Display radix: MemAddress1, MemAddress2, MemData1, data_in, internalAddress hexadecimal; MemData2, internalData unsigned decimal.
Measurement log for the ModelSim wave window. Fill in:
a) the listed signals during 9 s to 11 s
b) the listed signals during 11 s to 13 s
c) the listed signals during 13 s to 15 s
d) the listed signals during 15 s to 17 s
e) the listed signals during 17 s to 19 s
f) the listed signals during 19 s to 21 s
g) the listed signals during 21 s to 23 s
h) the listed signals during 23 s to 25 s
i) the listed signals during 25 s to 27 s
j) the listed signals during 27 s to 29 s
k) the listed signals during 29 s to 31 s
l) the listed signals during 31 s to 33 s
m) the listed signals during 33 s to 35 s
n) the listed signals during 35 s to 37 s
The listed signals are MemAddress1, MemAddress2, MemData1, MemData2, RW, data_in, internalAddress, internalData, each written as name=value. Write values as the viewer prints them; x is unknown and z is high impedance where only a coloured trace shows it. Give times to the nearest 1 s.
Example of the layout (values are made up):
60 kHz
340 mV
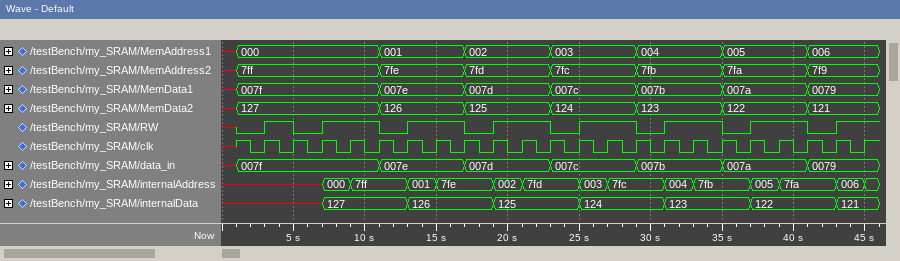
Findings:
MemAddress1=000, MemAddress2=7ff, MemData1=007f, MemData2=127, RW=1, data_in=007f, internalAddress=7ff, internalData=127
MemAddress1=001, MemAddress2=7fe, MemData1=007e, MemData2=126, RW=0, data_in=007e, internalAddress=7ff, internalData=127
MemAddress1=001, MemAddress2=7fe, MemData1=007e, MemData2=126, RW=1, data_in=007e, internalAddress=001, internalData=126
MemAddress1=001, MemAddress2=7fe, MemData1=007e, MemData2=126, RW=1, data_in=007e, internalAddress=7fe, internalData=126
MemAddress1=002, MemAddress2=7fd, MemData1=007d, MemData2=125, RW=0, data_in=007d, internalAddress=7fe, internalData=126
MemAddress1=002, MemAddress2=7fd, MemData1=007d, MemData2=125, RW=1, data_in=007d, internalAddress=002, internalData=125
MemAddress1=002, MemAddress2=7fd, MemData1=007d, MemData2=125, RW=1, data_in=007d, internalAddress=7fd, internalData=125
MemAddress1=003, MemAddress2=7fc, MemData1=007c, MemData2=124, RW=0, data_in=007c, internalAddress=7fd, internalData=125
MemAddress1=003, MemAddress2=7fc, MemData1=007c, MemData2=124, RW=1, data_in=007c, internalAddress=003, internalData=124
MemAddress1=003, MemAddress2=7fc, MemData1=007c, MemData2=124, RW=1, data_in=007c, internalAddress=7fc, internalData=124
MemAddress1=004, MemAddress2=7fb, MemData1=007b, MemData2=123, RW=0, data_in=007b, internalAddress=7fc, internalData=124
MemAddress1=004, MemAddress2=7fb, MemData1=007b, MemData2=123, RW=1, data_in=007b, internalAddress=004, internalData=123
MemAddress1=004, MemAddress2=7fb, MemData1=007b, MemData2=123, RW=1, data_in=007b, internalAddress=7fb, internalData=123
MemAddress1=005, MemAddress2=7fa, MemData1=007a, MemData2=122, RW=0, data_in=007a, internalAddress=7fb, internalData=123
